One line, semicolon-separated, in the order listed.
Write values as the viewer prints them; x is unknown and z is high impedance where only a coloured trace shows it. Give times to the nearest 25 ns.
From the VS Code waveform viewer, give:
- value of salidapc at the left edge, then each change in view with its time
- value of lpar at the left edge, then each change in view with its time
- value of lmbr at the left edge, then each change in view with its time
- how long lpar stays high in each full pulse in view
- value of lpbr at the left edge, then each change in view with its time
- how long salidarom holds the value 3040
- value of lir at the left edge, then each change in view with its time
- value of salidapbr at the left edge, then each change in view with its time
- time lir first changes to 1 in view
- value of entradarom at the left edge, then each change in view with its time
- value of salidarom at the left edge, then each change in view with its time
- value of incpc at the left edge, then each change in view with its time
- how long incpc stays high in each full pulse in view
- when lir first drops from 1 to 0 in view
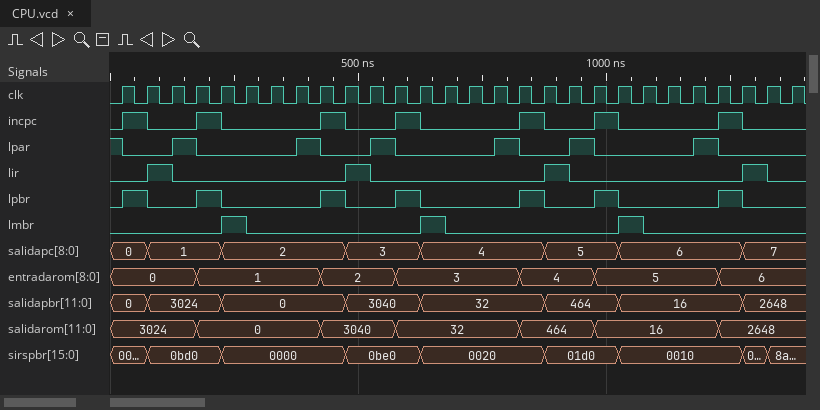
0, 1 at 75 ns, 2 at 225 ns, 3 at 475 ns, 4 at 625 ns, 5 at 875 ns, 6 at 1025 ns, 7 at 1275 ns; 1, 0 at 25 ns, 1 at 125 ns, 0 at 175 ns, 1 at 375 ns, 0 at 425 ns, 1 at 525 ns, 0 at 575 ns, 1 at 775 ns, 0 at 825 ns, 1 at 925 ns, 0 at 975 ns, 1 at 1175 ns, 0 at 1225 ns; 0, 1 at 225 ns, 0 at 275 ns, 1 at 625 ns, 0 at 675 ns, 1 at 1025 ns, 0 at 1075 ns; 50 ns, 50 ns, 50 ns, 50 ns, 50 ns, 50 ns; 0, 1 at 25 ns, 0 at 75 ns, 1 at 175 ns, 0 at 225 ns, 1 at 425 ns, 0 at 475 ns, 1 at 575 ns, 0 at 625 ns, 1 at 825 ns, 0 at 875 ns, 1 at 975 ns, 0 at 1025 ns, 1 at 1225 ns, 0 at 1275 ns; 150 ns; 0, 1 at 75 ns, 0 at 125 ns, 1 at 475 ns, 0 at 525 ns, 1 at 875 ns, 0 at 925 ns, 1 at 1275 ns, 0 at 1325 ns; 0, 3024 at 75 ns, 0 at 225 ns, 3040 at 475 ns, 32 at 625 ns, 464 at 875 ns, 16 at 1025 ns, 2648 at 1275 ns; 75 ns; 0, 1 at 175 ns, 2 at 425 ns, 3 at 575 ns, 4 at 825 ns, 5 at 975 ns, 6 at 1225 ns; 3024, 0 at 175 ns, 3040 at 425 ns, 32 at 575 ns, 464 at 825 ns, 16 at 975 ns, 2648 at 1225 ns; 0, 1 at 25 ns, 0 at 75 ns, 1 at 175 ns, 0 at 225 ns, 1 at 425 ns, 0 at 475 ns, 1 at 575 ns, 0 at 625 ns, 1 at 825 ns, 0 at 875 ns, 1 at 975 ns, 0 at 1025 ns, 1 at 1225 ns, 0 at 1275 ns; 50 ns, 50 ns, 50 ns, 50 ns, 50 ns, 50 ns, 50 ns; 125 ns
